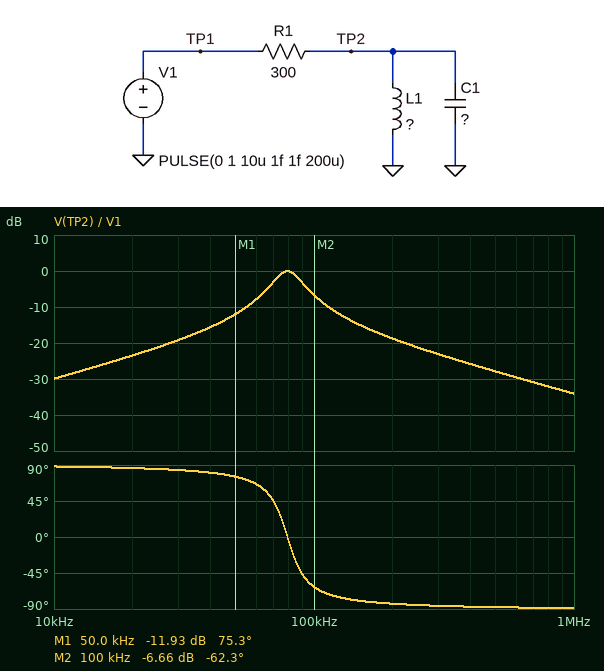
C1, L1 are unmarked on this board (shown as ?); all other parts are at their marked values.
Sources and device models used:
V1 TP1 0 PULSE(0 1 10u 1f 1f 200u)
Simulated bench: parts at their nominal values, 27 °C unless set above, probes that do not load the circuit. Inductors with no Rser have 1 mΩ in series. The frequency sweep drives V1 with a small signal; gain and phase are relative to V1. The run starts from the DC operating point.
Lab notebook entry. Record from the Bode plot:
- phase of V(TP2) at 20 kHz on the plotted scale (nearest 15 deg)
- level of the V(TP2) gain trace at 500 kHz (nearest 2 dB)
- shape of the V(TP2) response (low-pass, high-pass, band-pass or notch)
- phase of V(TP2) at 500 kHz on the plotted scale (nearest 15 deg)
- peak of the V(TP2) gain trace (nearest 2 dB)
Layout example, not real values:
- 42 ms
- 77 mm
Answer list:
- 90 deg
- -28 dB
- band-pass
- -90 deg
- 0 dB
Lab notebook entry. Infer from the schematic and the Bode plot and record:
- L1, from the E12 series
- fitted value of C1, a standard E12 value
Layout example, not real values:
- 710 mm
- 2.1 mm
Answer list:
- 150 µH
- 27 nF
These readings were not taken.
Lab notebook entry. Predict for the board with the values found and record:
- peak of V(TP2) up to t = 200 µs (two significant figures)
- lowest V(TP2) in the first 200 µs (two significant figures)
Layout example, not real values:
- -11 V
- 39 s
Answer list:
- 210 mV
- -140 mV
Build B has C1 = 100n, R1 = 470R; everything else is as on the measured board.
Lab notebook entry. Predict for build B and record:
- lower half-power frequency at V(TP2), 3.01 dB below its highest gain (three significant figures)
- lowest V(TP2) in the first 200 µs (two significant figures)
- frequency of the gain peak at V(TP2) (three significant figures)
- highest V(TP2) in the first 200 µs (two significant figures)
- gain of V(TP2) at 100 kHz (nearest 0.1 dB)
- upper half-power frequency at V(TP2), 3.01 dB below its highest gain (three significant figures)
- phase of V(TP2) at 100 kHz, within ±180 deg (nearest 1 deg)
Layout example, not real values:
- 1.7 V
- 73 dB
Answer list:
- 39.4 kHz
- -68 mV
- 41.1 kHz
- 77 mV
- -27.8 dB
- 42.8 kHz
- -88 deg
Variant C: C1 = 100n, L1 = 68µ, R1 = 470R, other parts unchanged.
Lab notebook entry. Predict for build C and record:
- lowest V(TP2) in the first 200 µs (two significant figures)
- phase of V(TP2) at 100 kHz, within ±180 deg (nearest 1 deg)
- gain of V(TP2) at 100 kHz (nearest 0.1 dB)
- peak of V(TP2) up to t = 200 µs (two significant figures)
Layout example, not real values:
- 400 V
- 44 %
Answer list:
- -49 mV
- -87 deg
- -25.4 dB
- 53 mV
